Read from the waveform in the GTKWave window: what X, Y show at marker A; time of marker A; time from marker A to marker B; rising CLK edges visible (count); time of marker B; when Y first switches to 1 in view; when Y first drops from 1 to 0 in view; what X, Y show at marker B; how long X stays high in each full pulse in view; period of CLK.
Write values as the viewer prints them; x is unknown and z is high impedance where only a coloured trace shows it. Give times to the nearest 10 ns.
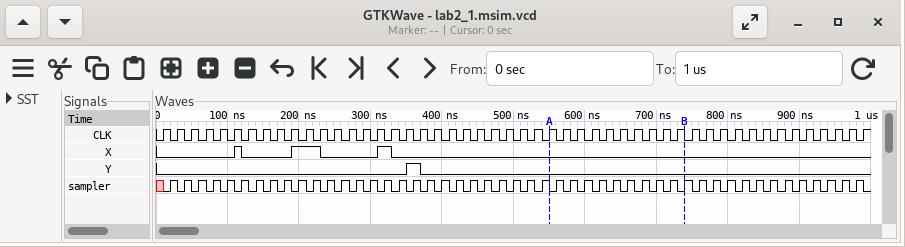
X=0, Y=0
550 ns
190 ns
50
740 ns
350 ns
370 ns
X=0, Y=0
10 ns, 40 ns, 20 ns
20 ns
